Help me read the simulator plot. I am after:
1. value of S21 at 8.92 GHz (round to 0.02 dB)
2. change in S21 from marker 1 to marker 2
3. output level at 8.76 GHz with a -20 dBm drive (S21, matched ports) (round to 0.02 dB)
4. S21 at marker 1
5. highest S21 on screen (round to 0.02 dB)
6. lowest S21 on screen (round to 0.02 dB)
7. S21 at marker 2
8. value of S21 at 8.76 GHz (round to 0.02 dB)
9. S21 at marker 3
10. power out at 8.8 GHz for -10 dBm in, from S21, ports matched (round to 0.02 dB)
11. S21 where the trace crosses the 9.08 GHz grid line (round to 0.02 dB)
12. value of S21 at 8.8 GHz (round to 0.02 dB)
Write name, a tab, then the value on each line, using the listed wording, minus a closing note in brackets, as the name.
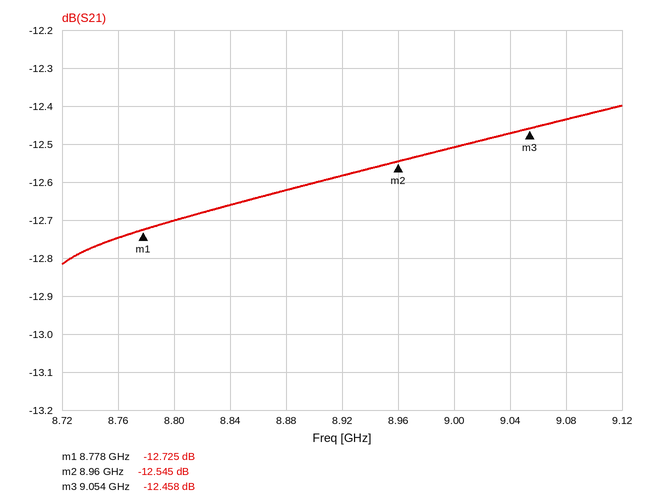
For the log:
value of S21 at 8.92 GHz	-12.58 dB
change in S21 from marker 1 to marker 2	0.180 dB
output level at 8.76 GHz with a -20 dBm drive (S21, matched ports)	-32.74 dBm
S21 at marker 1	-12.725 dB
highest S21 on screen	-12.40 dB
lowest S21 on screen	-12.82 dB
S21 at marker 2	-12.545 dB
value of S21 at 8.76 GHz	-12.74 dB
S21 at marker 3	-12.458 dB
power out at 8.8 GHz for -10 dBm in, from S21, ports matched	-22.70 dBm
S21 where the trace crosses the 9.08 GHz grid line	-12.44 dB
value of S21 at 8.8 GHz	-12.70 dB
